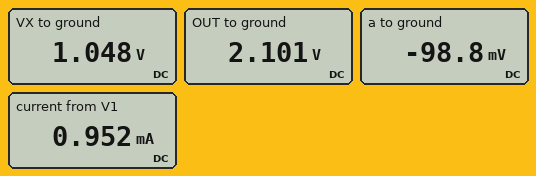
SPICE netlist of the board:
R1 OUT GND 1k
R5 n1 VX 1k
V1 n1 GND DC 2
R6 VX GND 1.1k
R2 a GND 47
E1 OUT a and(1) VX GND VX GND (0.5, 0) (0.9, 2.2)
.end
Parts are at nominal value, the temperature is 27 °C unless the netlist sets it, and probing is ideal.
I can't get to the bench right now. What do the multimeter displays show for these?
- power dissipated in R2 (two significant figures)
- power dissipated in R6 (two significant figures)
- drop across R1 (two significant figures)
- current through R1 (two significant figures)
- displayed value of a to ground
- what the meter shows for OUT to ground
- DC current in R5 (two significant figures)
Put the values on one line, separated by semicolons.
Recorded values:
210 µW; 1.0 mW; 2.1 V; 2.1 mA; -98.8 mV; 2.101 V; 950 µA
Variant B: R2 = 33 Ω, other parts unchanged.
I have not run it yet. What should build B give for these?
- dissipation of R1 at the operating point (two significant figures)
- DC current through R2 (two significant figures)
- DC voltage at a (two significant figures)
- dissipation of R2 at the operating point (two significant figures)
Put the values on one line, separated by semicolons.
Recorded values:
4.5 mW; 2.1 mA; -70 mV; 150 µW
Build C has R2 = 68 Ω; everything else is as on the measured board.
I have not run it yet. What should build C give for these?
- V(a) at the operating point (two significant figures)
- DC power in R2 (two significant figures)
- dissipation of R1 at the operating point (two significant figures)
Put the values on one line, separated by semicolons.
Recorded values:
-140 mV; 290 µW; 4.2 mW
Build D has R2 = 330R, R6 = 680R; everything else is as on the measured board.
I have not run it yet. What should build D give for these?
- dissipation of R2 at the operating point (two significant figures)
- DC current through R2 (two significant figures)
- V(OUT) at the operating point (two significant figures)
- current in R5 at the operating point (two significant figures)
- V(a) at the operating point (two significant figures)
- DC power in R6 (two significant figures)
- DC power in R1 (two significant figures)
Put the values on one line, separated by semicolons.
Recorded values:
540 µW; 1.3 mA; 1.3 V; 1.2 mA; -420 mV; 960 µW; 1.6 mW
